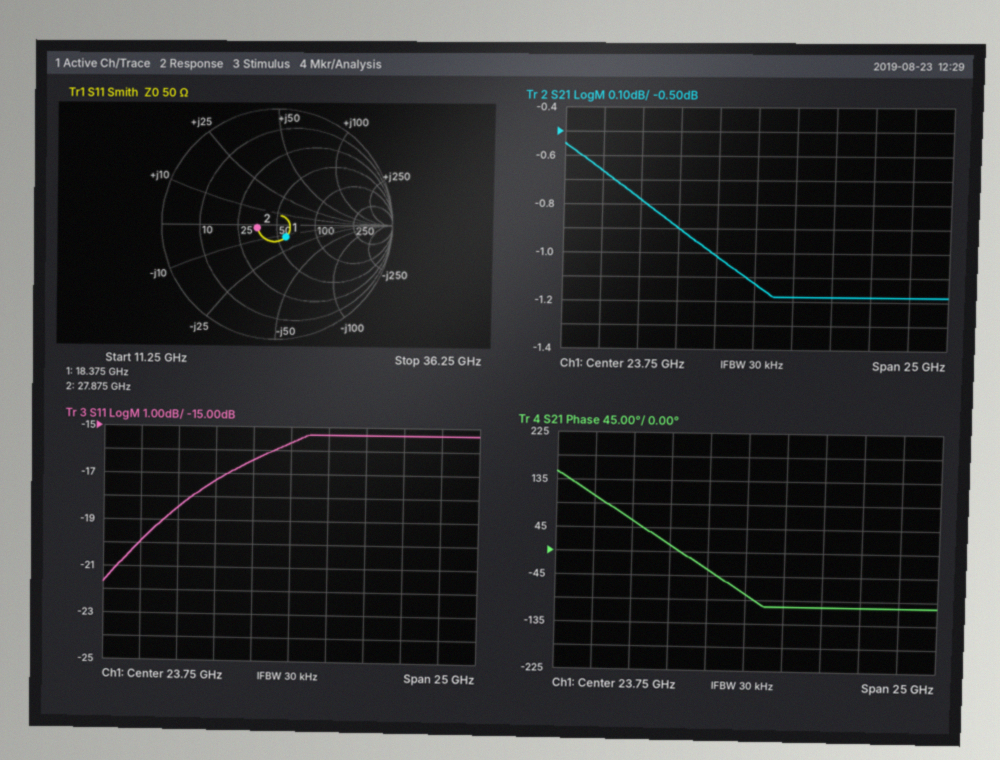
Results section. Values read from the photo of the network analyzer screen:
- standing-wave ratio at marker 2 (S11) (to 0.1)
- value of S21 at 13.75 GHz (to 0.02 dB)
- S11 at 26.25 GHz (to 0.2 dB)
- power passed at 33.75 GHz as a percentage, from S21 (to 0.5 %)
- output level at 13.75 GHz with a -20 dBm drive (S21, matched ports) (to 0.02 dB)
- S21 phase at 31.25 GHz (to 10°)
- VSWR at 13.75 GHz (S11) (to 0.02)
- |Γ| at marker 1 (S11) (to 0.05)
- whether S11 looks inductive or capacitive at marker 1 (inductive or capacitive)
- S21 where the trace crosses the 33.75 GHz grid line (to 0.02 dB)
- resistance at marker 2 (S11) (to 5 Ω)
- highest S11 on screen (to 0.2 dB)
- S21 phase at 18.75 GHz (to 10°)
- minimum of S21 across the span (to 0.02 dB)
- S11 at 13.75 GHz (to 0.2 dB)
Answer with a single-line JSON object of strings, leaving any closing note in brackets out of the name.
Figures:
{"standing-wave ratio at marker 2 (S11)": "1.4", "value of S21 at 13.75 GHz": "-0.66 dB", "S11 at 26.25 GHz": "-15.4 dB", "power passed at 33.75 GHz as a percentage, from S21": "76.0 %", "output level at 13.75 GHz with a -20 dBm drive (S21, matched ports)": "-20.66 dBm", "S21 phase at 31.25 GHz": "-100°", "VSWR at 13.75 GHz (S11)": "1.22", "|Γ| at marker 1 (S11)": "0.15", "whether S11 looks inductive or capacitive at marker 1": "capacitive", "S21 where the trace crosses the 33.75 GHz grid line": "-1.18 dB", "resistance at marker 2 (S11)": "35 Ω", "highest S11 on screen": "-15.4 dB", "S21 phase at 18.75 GHz": "10°", "minimum of S21 across the span": "-1.18 dB", "S11 at 13.75 GHz": "-20.0 dB"}
